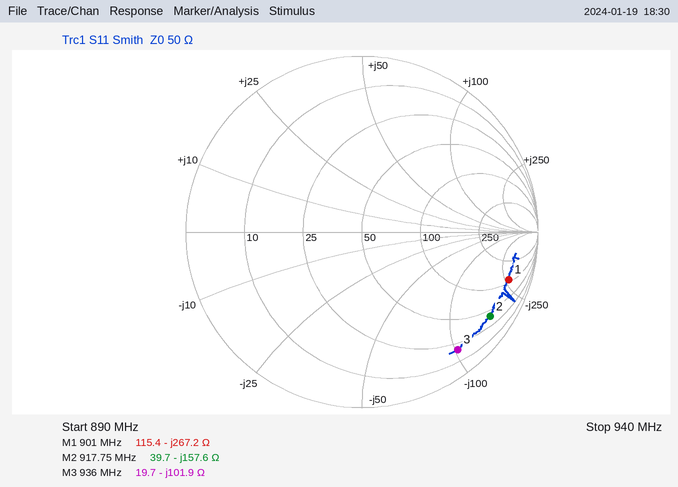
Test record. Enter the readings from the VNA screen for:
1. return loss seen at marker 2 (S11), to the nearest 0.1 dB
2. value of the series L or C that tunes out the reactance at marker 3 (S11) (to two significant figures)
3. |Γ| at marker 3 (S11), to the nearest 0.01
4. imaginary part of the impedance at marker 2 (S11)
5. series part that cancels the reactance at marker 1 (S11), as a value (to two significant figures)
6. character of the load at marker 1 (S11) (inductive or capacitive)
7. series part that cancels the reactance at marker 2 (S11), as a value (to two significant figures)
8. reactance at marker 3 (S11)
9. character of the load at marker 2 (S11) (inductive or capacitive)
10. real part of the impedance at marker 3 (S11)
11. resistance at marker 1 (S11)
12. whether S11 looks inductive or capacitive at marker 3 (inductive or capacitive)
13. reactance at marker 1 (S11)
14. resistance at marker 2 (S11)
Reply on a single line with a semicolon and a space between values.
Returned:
1.2 dB; 17 nH; 0.86; -157.6 Ω; 47 nH; capacitive; 27 nH; -101.9 Ω; capacitive; 19.7 Ω; 115.4 Ω; capacitive; -267.2 Ω; 39.7 Ω
